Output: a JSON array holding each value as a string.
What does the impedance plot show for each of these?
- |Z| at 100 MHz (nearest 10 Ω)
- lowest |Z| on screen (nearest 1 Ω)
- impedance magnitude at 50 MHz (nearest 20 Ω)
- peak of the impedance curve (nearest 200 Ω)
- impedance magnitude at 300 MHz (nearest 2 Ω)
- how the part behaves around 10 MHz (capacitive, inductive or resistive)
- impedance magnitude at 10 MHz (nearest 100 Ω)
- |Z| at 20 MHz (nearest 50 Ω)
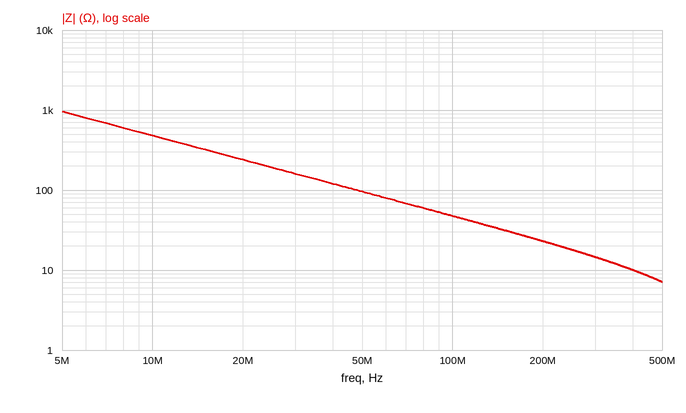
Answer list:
["50 Ω", "7 Ω", "100 Ω", "1.0 kΩ", "14 Ω", "capacitive", "500 Ω", "250 Ω"]
